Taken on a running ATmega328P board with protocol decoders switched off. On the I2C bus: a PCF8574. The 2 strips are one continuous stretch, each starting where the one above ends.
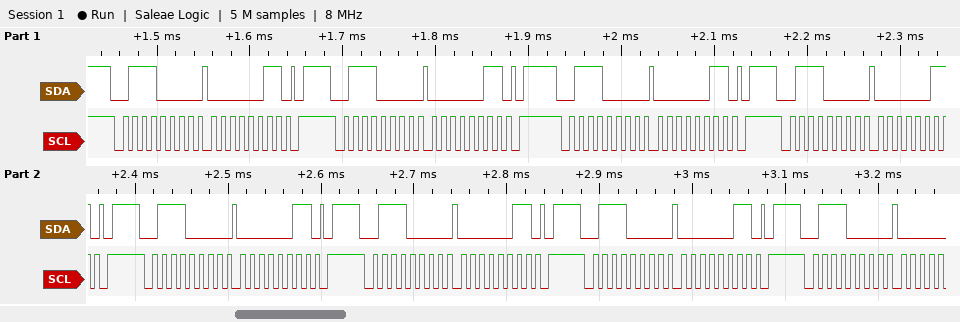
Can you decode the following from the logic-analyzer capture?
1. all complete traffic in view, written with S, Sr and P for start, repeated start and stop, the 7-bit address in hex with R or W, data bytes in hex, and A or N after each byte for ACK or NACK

S 38W A 03 A P S 38W A 03 A P S 38W A 03 A P S 38W A 03 A P S 38W A 03 A P S 38W A 03 A P S 38W A 03 A P S 38W A
